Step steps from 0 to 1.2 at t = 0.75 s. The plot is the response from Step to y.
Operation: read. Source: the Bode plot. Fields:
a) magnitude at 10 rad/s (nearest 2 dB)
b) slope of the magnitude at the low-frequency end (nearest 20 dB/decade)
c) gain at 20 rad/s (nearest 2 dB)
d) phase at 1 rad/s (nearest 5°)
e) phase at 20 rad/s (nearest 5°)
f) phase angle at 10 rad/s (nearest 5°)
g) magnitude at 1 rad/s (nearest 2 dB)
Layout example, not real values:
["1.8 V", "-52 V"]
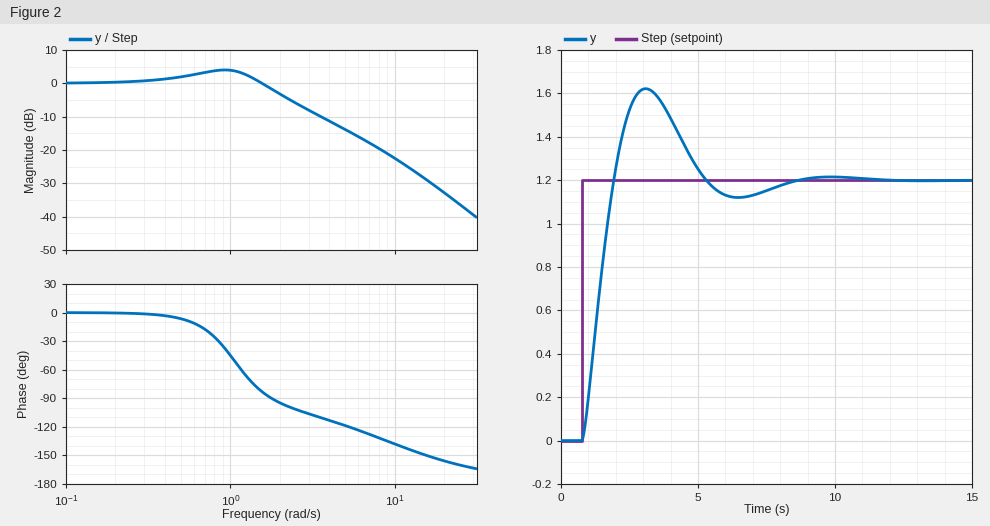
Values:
["-22 dB", "0 dB/decade", "-32 dB", "-45°", "-155°", "-140°", "4 dB"]
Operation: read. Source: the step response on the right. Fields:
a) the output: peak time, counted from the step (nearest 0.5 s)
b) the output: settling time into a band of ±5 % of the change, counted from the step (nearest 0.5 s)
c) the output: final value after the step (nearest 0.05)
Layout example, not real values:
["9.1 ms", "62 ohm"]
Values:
["2.5 s", "6.5 s", "1.20"]
